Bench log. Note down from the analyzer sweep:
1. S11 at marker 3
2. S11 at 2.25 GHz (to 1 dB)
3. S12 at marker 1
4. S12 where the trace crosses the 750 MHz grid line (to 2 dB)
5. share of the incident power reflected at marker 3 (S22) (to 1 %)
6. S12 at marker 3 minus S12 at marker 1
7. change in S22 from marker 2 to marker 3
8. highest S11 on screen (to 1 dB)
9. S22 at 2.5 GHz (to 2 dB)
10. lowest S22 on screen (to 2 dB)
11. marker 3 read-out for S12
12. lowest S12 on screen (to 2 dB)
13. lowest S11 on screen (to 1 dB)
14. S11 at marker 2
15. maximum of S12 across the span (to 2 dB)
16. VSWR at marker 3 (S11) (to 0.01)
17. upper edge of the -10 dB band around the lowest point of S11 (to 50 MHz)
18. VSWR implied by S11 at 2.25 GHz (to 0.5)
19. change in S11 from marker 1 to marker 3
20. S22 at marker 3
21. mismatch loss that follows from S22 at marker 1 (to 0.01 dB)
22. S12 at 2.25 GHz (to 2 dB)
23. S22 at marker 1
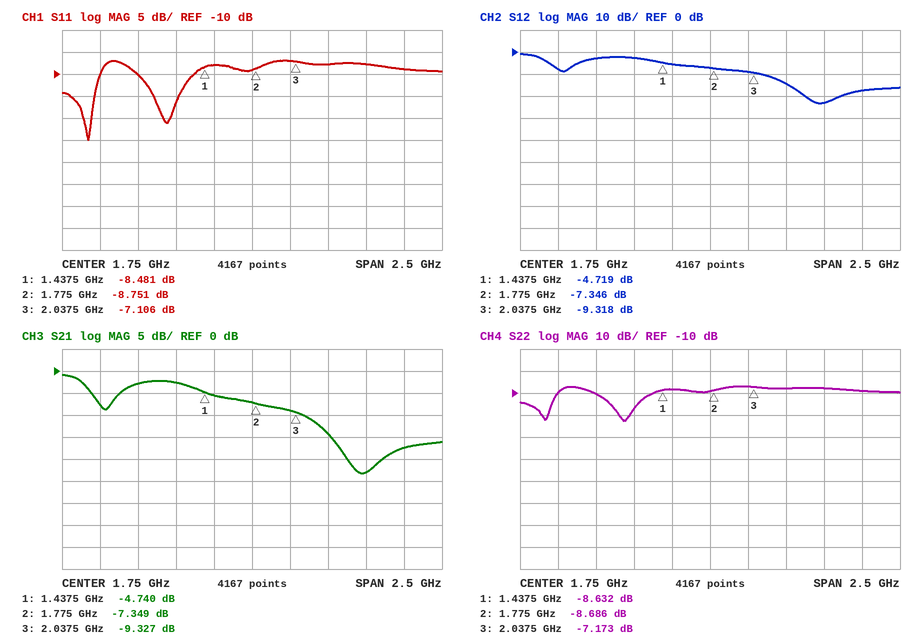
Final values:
-7.106 dB
-8 dB
-4.719 dB
-8 dB
19 %
-4.599 dB
1.513 dB
-7 dB
-8 dB
-22 dB
-9.318 dB
-24 dB
-25 dB
-8.751 dB
0 dB
2.58
750 MHz
2.5
1.375 dB
-7.173 dB
0.64 dB
-14 dB
-8.632 dB
